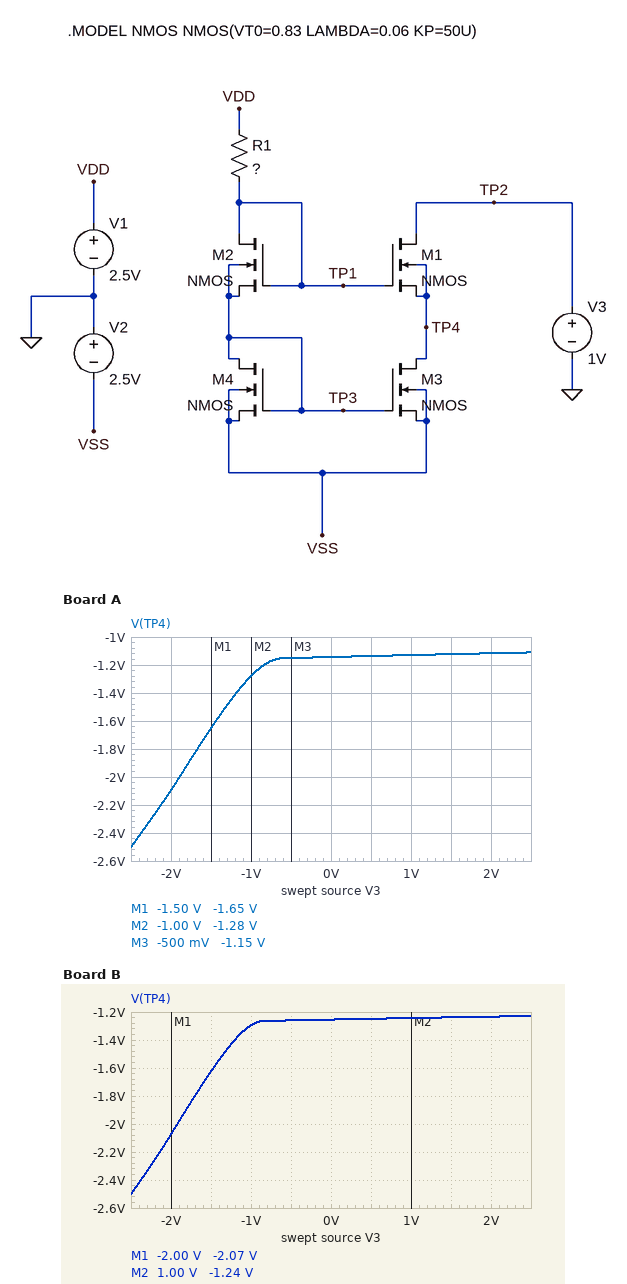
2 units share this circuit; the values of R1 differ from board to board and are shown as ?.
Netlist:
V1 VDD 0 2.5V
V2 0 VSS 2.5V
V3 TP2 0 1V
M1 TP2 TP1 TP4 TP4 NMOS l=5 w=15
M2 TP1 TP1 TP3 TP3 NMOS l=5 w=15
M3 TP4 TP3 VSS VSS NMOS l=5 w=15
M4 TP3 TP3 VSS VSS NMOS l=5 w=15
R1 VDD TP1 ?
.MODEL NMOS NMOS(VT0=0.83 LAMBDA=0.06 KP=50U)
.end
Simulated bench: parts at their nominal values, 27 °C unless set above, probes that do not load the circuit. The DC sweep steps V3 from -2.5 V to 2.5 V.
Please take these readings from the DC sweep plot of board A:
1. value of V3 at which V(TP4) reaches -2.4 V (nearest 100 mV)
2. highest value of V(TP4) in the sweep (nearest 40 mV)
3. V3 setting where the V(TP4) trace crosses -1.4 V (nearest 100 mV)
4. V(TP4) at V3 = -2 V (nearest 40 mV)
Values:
-2.4 V
-1.12 V
-1.2 V
-2.08 V
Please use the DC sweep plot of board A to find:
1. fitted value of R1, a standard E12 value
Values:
100 kΩ
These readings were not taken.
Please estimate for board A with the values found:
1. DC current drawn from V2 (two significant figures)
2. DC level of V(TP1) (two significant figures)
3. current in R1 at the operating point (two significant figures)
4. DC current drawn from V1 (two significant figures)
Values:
46 µA
220 mV
23 µA
23 µA
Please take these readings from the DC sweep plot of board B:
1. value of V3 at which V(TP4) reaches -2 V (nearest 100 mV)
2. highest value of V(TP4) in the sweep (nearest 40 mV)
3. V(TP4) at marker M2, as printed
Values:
-1.9 V
-1.24 V
-1.24 V
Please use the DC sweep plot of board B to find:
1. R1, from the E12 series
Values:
180 kΩ
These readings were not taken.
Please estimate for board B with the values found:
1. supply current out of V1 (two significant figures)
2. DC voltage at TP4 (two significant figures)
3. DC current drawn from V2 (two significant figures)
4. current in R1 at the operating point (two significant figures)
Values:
14 µA
-1.2 V
28 µA
14 µA
